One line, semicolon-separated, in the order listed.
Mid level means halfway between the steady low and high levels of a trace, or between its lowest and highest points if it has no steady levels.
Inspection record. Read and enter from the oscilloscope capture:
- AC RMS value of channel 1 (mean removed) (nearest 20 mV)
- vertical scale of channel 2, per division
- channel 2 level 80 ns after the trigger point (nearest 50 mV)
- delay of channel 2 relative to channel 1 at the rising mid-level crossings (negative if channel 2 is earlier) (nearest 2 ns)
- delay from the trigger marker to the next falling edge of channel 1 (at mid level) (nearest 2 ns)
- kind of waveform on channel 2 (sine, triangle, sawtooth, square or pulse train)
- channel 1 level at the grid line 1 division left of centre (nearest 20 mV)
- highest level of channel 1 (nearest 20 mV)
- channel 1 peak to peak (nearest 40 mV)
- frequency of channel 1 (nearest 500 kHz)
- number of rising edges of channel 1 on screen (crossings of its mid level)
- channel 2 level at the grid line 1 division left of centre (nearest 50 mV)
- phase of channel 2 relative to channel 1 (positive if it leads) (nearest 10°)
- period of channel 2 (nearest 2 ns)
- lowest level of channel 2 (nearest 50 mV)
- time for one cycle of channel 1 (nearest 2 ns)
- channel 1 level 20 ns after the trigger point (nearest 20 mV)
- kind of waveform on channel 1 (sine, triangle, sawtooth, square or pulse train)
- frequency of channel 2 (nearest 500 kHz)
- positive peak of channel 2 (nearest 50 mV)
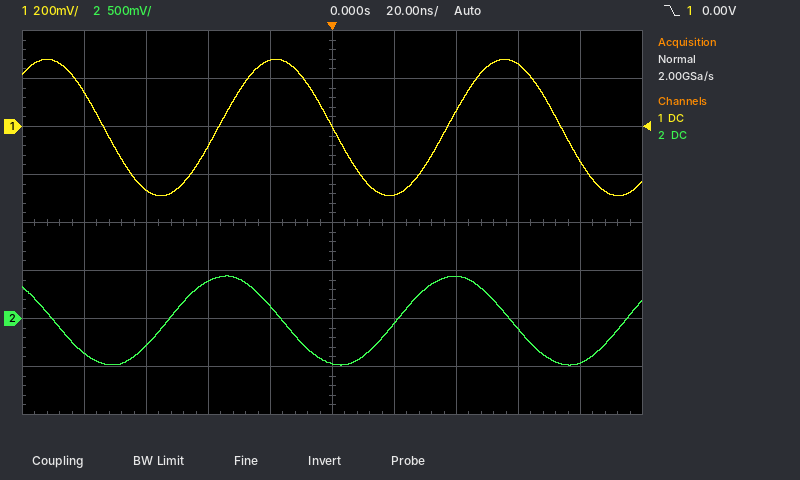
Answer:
200 mV; 500 mV; -450 mV; -16 ns; 74 ns; sine; 280 mV; 280 mV; 560 mV; 13.5 MHz; 2; 150 mV; +80°; 74 ns; -500 mV; 74 ns; -280 mV; sine; 13.5 MHz; 450 mV
